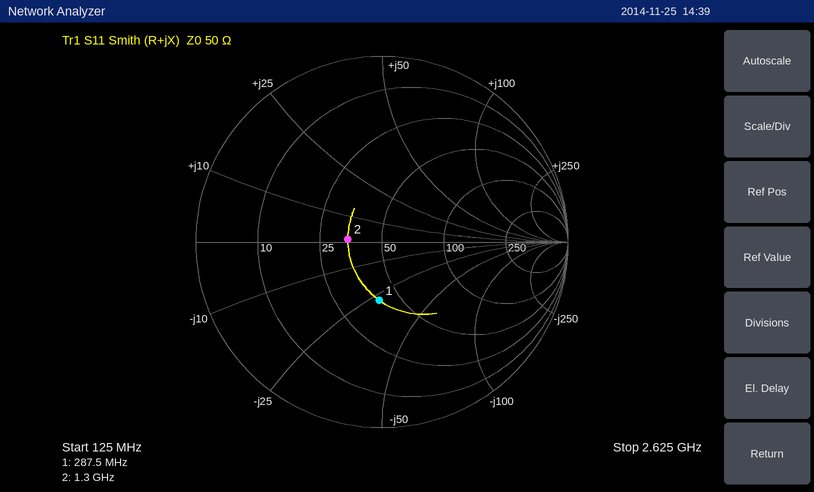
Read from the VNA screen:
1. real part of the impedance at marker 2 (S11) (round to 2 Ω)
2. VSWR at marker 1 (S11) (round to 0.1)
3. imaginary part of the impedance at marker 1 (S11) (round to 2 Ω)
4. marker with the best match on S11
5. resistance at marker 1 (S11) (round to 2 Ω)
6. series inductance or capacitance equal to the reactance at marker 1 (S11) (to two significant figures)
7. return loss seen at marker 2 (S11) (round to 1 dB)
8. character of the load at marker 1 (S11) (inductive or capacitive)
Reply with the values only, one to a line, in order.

34 Ω
1.9
-28 Ω
marker 2
40 Ω
20 pF
15 dB
capacitive
